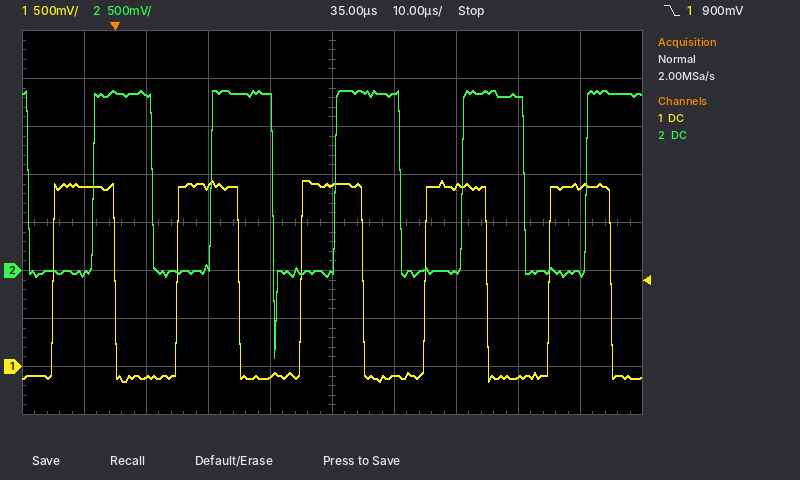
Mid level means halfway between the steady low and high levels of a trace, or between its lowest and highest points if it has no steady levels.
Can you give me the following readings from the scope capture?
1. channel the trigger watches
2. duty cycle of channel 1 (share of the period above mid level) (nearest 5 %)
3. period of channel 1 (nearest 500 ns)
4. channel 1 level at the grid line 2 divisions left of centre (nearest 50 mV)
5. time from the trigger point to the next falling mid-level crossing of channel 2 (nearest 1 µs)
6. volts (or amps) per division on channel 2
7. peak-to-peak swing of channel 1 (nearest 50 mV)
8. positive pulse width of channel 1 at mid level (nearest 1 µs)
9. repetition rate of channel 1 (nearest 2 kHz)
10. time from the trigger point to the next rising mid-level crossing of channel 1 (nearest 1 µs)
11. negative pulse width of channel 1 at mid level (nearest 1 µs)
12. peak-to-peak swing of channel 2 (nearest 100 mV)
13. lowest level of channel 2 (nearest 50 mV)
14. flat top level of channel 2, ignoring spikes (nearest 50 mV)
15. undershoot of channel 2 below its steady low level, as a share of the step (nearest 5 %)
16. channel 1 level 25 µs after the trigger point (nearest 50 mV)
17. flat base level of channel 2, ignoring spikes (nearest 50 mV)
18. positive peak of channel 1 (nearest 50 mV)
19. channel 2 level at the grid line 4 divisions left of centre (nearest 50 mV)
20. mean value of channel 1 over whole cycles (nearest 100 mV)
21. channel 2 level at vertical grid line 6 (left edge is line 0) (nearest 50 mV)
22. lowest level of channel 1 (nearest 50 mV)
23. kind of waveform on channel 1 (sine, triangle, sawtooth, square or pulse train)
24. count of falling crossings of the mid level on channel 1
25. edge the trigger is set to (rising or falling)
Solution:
channel 1
50 %
20.0 µs
1.90 V
6 µs
500 mV
2.10 V
10 µs
50 kHz
10 µs
10 µs
2.80 V
-900 mV
1.85 V
50 %
-100 mV
0 mV
1.95 V
-50 mV
900 mV
1.85 V
-150 mV
square
5
falling
